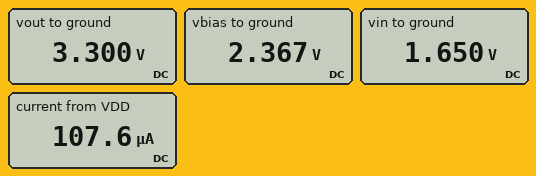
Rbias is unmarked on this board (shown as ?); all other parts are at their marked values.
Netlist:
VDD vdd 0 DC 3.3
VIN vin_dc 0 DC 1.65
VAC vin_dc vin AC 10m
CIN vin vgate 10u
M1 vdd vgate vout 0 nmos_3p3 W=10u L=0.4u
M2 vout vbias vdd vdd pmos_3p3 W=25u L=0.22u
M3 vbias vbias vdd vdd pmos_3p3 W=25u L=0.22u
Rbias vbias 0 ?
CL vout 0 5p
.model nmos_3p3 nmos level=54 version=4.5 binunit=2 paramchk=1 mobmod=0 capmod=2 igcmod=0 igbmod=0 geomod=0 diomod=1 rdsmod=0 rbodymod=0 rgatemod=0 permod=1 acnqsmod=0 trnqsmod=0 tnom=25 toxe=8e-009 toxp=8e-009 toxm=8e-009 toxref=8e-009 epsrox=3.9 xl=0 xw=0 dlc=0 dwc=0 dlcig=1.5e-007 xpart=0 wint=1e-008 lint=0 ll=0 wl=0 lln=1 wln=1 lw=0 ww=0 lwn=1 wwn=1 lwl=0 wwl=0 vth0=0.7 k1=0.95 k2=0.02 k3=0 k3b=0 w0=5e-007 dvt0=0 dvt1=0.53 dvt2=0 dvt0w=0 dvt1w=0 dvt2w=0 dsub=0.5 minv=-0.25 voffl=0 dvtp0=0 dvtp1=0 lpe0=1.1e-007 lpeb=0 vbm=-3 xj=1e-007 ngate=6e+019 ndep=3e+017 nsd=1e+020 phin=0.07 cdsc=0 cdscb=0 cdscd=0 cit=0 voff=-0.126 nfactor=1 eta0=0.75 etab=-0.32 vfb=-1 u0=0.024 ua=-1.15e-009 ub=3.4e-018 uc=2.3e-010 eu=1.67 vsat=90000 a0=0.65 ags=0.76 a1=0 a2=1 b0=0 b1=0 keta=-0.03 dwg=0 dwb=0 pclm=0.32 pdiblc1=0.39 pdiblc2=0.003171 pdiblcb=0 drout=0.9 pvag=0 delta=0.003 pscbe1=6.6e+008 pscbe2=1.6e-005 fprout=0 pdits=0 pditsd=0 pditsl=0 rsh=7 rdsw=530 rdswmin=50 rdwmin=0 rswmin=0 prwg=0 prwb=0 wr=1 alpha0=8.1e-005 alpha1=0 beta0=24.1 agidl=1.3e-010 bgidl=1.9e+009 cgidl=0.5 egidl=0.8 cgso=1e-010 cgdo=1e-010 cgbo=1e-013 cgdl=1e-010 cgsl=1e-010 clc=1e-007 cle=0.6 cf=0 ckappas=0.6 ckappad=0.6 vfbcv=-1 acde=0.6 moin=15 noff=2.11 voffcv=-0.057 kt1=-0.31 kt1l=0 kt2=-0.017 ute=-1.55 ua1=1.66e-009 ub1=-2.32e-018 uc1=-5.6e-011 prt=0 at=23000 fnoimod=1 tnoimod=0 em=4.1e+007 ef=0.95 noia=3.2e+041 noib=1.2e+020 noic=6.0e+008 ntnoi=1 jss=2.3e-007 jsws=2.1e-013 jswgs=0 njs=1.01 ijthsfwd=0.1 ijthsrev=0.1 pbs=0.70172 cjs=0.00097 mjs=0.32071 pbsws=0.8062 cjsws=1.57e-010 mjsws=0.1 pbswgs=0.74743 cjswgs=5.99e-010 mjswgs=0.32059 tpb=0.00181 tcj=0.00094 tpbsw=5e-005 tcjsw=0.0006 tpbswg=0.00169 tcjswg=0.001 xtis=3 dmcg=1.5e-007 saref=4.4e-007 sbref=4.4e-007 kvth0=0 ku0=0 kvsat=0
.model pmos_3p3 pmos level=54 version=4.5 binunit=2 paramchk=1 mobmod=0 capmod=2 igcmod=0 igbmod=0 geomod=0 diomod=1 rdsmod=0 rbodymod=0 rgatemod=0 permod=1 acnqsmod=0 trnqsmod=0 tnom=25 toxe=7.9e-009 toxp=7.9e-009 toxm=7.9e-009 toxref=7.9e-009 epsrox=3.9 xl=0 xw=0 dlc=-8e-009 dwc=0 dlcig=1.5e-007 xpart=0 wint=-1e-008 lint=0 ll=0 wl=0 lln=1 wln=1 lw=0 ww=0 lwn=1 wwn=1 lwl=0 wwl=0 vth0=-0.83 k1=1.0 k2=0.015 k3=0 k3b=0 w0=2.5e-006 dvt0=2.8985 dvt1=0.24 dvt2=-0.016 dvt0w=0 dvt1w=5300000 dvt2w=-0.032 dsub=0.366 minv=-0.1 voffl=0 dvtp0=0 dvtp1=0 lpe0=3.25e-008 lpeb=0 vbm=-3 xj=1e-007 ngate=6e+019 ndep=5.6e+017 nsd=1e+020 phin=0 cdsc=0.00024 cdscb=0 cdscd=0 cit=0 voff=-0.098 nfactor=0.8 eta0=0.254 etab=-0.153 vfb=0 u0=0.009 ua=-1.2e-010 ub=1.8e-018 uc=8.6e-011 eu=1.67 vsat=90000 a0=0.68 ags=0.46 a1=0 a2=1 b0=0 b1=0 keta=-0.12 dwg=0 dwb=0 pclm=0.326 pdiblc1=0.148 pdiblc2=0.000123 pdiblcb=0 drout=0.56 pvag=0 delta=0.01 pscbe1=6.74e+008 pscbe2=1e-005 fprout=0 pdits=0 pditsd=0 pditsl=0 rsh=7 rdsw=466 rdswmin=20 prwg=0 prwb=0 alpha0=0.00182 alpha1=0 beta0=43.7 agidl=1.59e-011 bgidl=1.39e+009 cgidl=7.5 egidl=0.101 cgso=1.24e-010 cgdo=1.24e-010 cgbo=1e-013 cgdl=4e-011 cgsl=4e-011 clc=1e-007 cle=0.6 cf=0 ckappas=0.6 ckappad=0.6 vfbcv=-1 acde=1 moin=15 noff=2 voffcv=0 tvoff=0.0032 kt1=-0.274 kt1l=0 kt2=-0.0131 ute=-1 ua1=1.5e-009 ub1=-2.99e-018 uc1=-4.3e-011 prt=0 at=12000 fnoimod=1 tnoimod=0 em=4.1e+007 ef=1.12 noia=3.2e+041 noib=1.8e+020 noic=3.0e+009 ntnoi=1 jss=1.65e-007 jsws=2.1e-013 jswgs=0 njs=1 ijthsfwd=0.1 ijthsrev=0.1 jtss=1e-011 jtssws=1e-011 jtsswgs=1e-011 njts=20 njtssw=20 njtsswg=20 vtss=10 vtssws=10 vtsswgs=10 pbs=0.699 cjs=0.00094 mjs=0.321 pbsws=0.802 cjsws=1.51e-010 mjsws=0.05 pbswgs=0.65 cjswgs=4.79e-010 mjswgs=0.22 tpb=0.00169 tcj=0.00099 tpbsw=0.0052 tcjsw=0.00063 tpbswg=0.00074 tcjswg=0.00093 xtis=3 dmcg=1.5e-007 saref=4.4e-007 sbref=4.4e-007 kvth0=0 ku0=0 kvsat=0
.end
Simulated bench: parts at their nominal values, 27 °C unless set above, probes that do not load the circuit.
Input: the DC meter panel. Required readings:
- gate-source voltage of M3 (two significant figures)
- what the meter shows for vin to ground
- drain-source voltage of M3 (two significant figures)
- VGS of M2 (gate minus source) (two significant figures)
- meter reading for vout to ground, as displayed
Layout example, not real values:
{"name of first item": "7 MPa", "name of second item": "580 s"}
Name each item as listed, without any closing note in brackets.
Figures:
{"gate-source voltage of M3": "-930 mV", "what the meter shows for vin to ground": "1.650 V", "drain-source voltage of M3": "-930 mV", "VGS of M2 (gate minus source)": "-930 mV", "meter reading for vout to ground, as displayed": "3.300 V"}
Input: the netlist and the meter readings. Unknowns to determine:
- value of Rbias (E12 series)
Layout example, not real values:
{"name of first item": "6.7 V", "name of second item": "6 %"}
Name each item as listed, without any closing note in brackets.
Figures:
{"value of Rbias": "22 kΩ"}
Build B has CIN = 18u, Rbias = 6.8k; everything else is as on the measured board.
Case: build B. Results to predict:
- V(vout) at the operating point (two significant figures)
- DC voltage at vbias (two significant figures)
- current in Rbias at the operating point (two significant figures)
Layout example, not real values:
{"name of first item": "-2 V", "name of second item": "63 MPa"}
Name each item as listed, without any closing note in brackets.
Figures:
{"V(vout) at the operating point": "3.3 V", "DC voltage at vbias": "2.2 V", "current in Rbias at the operating point": "320 µA"}
